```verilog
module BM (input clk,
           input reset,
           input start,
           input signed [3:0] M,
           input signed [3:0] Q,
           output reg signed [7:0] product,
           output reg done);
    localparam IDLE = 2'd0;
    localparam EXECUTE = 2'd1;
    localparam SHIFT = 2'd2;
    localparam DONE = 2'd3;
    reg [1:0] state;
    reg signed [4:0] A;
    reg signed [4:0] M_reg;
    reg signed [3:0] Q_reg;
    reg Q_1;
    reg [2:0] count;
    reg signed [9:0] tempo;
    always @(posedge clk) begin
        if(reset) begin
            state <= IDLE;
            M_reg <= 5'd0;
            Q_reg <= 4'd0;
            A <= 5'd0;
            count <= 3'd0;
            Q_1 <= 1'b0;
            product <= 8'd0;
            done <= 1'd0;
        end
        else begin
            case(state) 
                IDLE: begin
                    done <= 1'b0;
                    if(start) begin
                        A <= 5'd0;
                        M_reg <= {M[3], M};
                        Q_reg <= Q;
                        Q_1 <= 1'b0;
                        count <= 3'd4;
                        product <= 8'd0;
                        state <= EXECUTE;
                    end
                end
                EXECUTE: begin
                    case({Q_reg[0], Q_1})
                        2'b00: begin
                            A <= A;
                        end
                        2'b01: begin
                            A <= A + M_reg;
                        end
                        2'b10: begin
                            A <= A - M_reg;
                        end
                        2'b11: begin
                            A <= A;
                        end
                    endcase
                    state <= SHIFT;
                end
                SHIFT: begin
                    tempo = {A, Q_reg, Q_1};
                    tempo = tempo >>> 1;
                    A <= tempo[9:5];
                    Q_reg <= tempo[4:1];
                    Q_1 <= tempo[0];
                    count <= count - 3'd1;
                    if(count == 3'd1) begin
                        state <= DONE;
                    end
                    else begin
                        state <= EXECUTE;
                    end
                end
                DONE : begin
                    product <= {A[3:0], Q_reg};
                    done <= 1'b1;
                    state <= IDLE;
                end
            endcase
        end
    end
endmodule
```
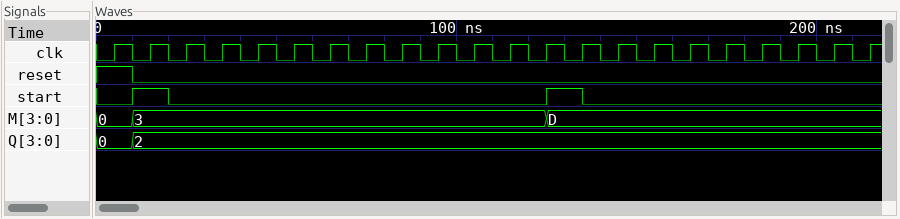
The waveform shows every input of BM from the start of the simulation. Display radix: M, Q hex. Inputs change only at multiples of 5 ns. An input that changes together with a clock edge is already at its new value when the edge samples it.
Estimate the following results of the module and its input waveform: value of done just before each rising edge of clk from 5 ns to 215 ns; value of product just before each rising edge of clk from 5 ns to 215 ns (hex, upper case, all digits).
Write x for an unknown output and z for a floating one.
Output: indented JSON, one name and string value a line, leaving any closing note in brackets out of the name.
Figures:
{
  "value of done just before each rising edge of clk from 5 ns to 215 ns": "x 0 0 0 0 0 0 0 0 0 0 1 0 0 0 0 0 0 0 0 0 0",
  "value of product just before each rising edge of clk from 5 ns to 215 ns": "x, 00, 00, 00, 00, 00, 00, 00, 00, 00, 00, 06, 06, 00, 00, 00, 00, 00, 00, 00, 00, 00"
}
